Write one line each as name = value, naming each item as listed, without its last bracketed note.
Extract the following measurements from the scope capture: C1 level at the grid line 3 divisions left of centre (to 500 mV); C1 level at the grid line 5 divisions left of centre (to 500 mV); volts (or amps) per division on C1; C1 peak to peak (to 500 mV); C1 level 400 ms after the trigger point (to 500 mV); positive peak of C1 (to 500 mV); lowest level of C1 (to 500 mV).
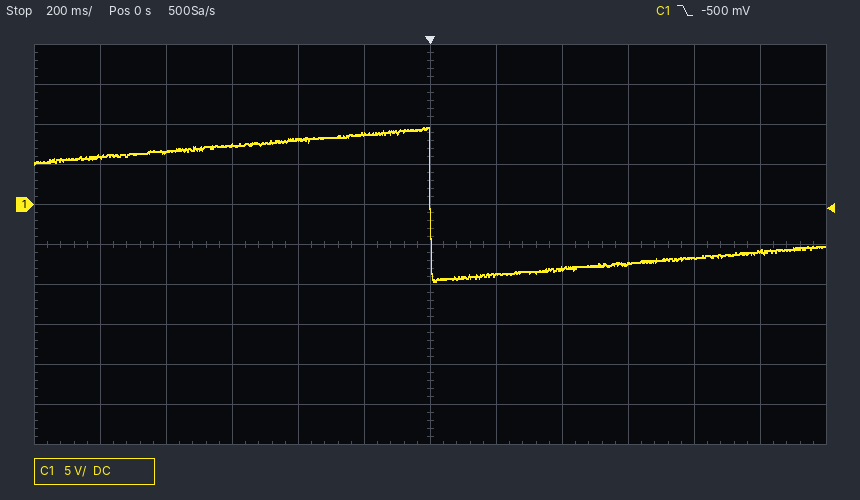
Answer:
C1 level at the grid line 3 divisions left of centre = 7.5 V
C1 level at the grid line 5 divisions left of centre = 6.0 V
volts (or amps) per division on C1 = 5 V
C1 peak to peak = 19.0 V
C1 level 400 ms after the trigger point = -8.0 V
positive peak of C1 = 9.5 V
lowest level of C1 = -9.5 V
